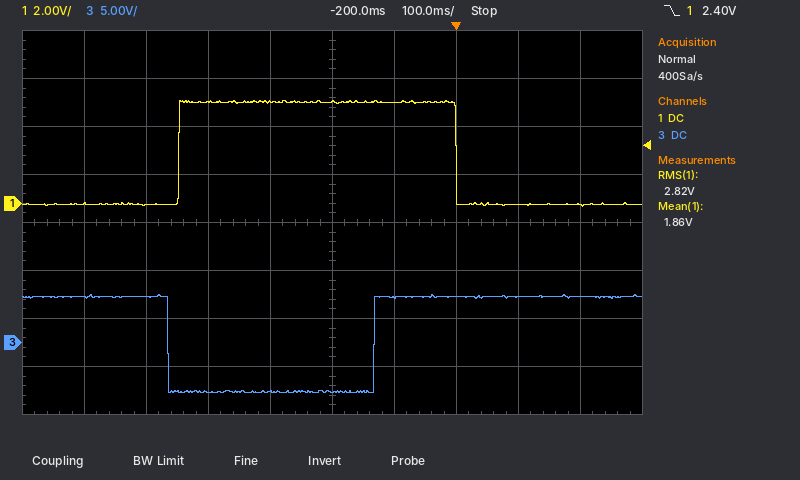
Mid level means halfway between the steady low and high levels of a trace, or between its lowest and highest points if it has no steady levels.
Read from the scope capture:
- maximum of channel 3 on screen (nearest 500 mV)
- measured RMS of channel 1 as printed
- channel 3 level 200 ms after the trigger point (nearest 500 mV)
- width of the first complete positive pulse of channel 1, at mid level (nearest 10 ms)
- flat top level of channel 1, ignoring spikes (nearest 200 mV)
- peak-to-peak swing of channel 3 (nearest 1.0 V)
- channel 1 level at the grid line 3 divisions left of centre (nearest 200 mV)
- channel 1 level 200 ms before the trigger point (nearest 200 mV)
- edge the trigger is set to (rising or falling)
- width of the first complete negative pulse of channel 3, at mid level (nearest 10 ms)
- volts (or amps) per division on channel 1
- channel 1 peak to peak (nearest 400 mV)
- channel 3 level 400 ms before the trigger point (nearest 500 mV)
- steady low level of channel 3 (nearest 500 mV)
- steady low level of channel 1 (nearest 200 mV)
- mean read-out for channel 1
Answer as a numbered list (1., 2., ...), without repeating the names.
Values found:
1. 5.0 V
2. 2.82 V
3. 5.0 V
4. 450 ms
5. 4.2 V
6. 10.0 V
7. 0.0 V
8. 4.2 V
9. falling
10. 330 ms
11. 2 V
12. 4.4 V
13. -5.0 V
14. -5.0 V
15. 0.0 V
16. 1.86 V
